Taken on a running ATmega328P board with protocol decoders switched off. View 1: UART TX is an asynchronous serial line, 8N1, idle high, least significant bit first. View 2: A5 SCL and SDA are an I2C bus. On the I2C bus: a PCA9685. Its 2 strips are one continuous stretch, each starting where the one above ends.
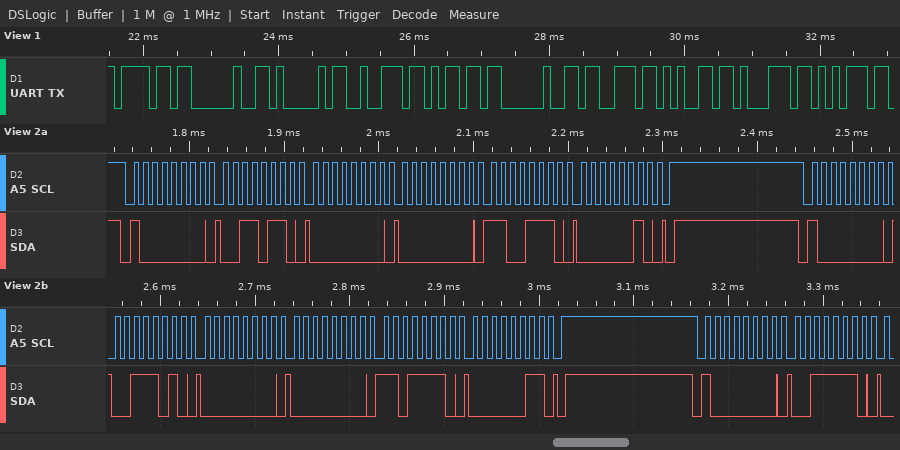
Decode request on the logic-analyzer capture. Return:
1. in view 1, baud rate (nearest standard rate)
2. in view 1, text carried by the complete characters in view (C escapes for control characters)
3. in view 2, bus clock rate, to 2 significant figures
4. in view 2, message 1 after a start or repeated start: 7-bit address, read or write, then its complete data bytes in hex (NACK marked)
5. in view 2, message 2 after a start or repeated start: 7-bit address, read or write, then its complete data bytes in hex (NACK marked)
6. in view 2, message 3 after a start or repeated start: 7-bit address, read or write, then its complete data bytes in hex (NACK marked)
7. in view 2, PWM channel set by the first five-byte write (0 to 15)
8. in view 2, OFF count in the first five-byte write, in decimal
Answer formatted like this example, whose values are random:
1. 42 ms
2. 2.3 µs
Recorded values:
1. 9600 baud
2. "o Arm sequ"
3. 100 kHz
4. 0x40 write: 36 00 00 CE 02
5. 0x40 write: 3A 00 00 DE 03
6. 0x40 write: 3E
7. 12
8. 718
